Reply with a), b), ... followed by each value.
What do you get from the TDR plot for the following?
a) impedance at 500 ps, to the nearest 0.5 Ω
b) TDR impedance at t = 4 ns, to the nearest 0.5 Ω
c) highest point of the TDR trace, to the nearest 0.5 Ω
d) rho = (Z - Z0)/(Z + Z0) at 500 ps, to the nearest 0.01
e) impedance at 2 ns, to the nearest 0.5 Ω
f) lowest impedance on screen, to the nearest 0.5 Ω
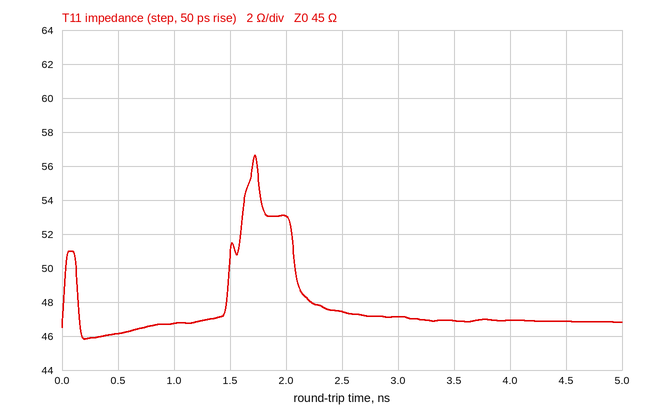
a) 46.0 Ω
b) 47.0 Ω
c) 56.5 Ω
d) +0.01
e) 53.0 Ω
f) 46.0 Ω
